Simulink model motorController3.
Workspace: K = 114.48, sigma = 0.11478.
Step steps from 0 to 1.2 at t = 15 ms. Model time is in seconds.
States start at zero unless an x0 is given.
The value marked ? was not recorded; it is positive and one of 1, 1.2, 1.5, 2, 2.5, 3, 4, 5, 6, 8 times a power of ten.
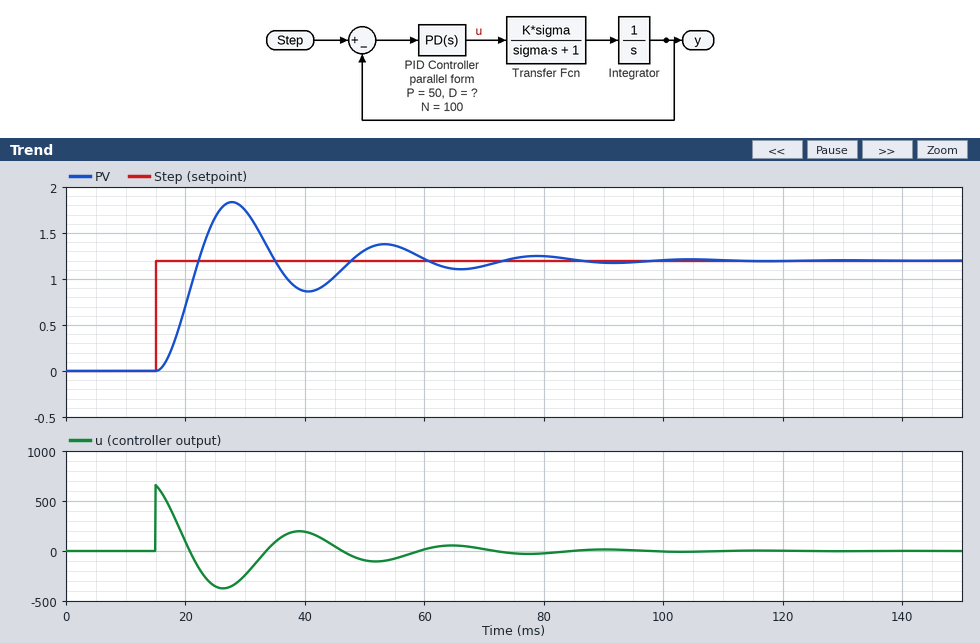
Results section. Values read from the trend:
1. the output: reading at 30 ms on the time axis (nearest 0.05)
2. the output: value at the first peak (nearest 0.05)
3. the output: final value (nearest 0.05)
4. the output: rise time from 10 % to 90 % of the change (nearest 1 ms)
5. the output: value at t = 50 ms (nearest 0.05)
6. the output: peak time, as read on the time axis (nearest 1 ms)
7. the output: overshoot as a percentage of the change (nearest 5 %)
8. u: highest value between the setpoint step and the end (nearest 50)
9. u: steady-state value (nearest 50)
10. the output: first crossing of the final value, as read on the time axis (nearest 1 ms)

1.75
1.85
1.20
5 ms
1.30
28 ms
55 %
650
0
22 ms
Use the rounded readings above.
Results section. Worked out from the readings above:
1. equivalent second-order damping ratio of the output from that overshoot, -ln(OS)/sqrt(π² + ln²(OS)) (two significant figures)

0.19
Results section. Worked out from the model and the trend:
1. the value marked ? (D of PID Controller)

5
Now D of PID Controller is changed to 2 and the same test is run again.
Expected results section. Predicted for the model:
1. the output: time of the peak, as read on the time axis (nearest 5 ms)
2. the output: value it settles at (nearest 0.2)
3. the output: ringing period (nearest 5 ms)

35 ms
1.2
40 ms
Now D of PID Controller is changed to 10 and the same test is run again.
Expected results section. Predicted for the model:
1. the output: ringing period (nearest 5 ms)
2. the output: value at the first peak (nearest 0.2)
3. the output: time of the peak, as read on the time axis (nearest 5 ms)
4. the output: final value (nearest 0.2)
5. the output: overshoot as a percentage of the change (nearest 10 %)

20 ms
2.0
25 ms
1.2
60 %
